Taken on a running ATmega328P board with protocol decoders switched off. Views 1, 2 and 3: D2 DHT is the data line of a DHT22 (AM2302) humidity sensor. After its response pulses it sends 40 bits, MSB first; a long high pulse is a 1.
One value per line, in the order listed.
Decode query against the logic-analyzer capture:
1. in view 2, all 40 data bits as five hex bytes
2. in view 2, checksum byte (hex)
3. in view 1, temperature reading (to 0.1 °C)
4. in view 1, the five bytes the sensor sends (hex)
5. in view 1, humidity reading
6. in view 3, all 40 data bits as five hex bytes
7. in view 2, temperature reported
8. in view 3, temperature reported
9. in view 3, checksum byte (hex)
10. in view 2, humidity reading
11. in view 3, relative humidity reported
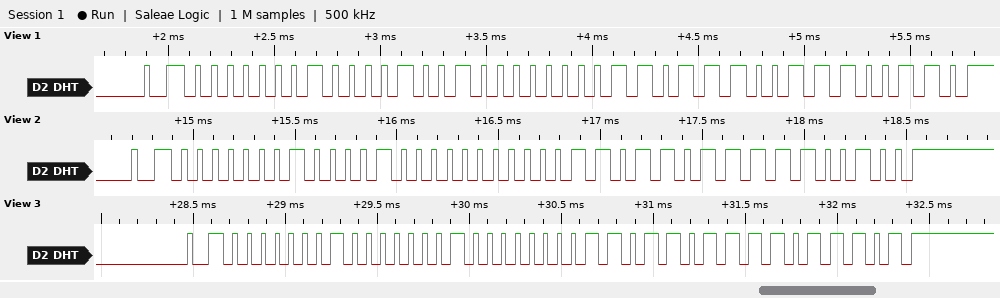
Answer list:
01 08 00 DB E4
0xE4
22.0 °C
01 09 00 DC E6
26.5 %
01 01 00 DB DD
21.9 °C
21.9 °C
0xDD
26.4 %
25.7 %
